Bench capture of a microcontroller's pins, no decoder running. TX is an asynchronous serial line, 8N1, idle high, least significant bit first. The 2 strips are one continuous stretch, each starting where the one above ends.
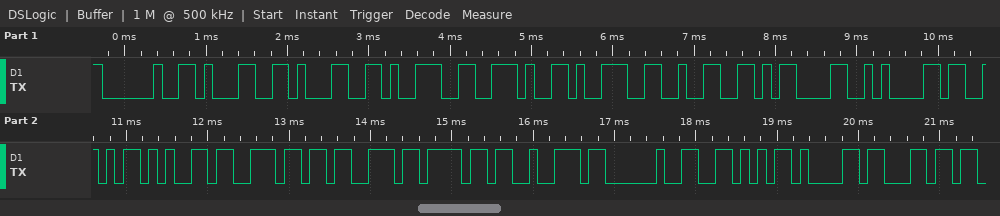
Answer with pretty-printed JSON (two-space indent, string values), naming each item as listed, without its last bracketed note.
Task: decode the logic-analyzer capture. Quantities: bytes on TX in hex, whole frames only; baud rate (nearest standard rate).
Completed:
{
  "bytes on TX in hex, whole frames only": "0x20 0x31 0x31 0x39 0x2E 0x39 0x32 0x0D 0x0A 0x53 0x65 0x6E 0x73 0x6F 0x72 0x20 0x56 0x61 0x6C",
  "baud rate": "9600 baud"
}
